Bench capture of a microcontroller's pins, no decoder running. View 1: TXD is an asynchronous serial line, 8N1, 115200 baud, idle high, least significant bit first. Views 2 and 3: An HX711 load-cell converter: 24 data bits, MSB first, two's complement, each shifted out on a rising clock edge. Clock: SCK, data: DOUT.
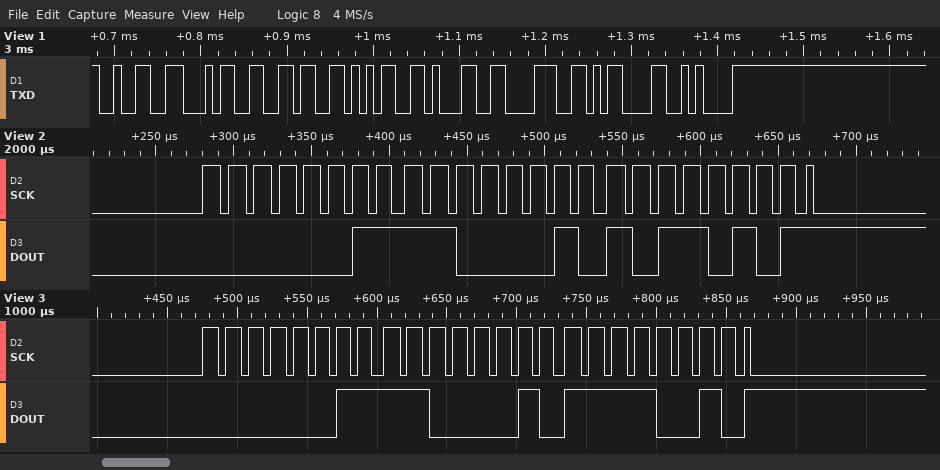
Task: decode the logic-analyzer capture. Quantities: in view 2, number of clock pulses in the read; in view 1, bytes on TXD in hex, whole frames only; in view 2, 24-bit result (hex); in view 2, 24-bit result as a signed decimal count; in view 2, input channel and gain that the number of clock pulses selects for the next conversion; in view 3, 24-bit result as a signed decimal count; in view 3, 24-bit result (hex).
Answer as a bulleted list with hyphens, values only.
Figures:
- 25
- 32 34 36 35 31 38 0D 0A
- 0x03C2B5
- 246453
- channel A, gain 128
- 246514
- 0x03C2F2
